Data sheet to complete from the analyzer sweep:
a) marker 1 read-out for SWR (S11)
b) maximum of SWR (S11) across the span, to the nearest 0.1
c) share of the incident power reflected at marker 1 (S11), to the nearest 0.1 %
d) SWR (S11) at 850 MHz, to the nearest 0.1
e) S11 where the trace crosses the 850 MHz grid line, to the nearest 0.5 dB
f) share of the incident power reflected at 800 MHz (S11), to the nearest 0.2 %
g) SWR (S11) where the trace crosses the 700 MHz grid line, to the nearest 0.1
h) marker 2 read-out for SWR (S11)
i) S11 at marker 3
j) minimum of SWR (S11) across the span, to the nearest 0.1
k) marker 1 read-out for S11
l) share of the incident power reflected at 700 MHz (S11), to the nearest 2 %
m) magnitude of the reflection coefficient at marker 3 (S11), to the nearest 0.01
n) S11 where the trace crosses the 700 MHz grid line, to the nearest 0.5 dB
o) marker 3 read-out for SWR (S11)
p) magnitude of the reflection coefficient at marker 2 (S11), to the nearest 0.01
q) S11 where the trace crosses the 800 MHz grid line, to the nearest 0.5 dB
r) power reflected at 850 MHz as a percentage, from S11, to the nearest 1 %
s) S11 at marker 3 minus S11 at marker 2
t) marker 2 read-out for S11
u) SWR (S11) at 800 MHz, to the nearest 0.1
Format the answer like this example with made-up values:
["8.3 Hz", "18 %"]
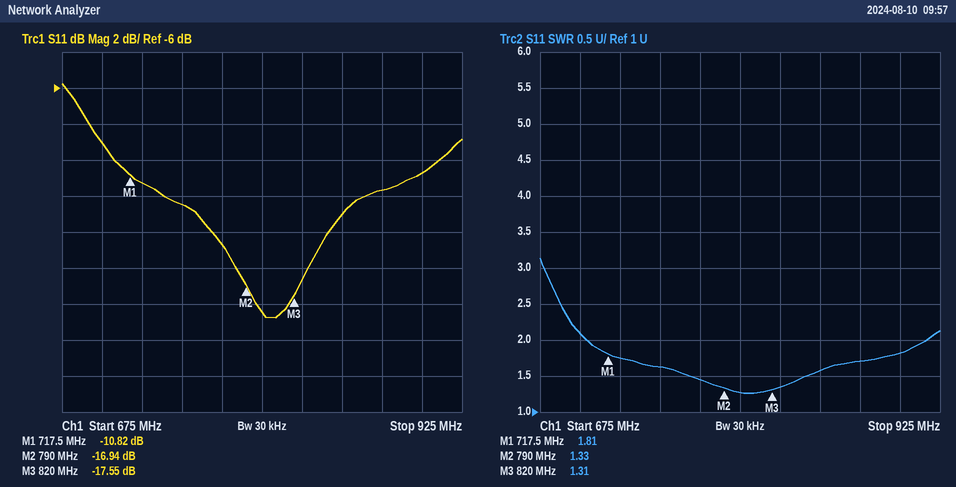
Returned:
["1.81", "3.1", "8.3 %", "1.6", "-13.0 dB", "1.4 %", "2.1", "1.33", "-17.55 dB", "1.3", "-10.82 dB", "12 %", "0.13", "-9.0 dB", "1.31", "0.14", "-18.5 dB", "5 %", "-0.61 dB", "-16.94 dB", "1.3"]
